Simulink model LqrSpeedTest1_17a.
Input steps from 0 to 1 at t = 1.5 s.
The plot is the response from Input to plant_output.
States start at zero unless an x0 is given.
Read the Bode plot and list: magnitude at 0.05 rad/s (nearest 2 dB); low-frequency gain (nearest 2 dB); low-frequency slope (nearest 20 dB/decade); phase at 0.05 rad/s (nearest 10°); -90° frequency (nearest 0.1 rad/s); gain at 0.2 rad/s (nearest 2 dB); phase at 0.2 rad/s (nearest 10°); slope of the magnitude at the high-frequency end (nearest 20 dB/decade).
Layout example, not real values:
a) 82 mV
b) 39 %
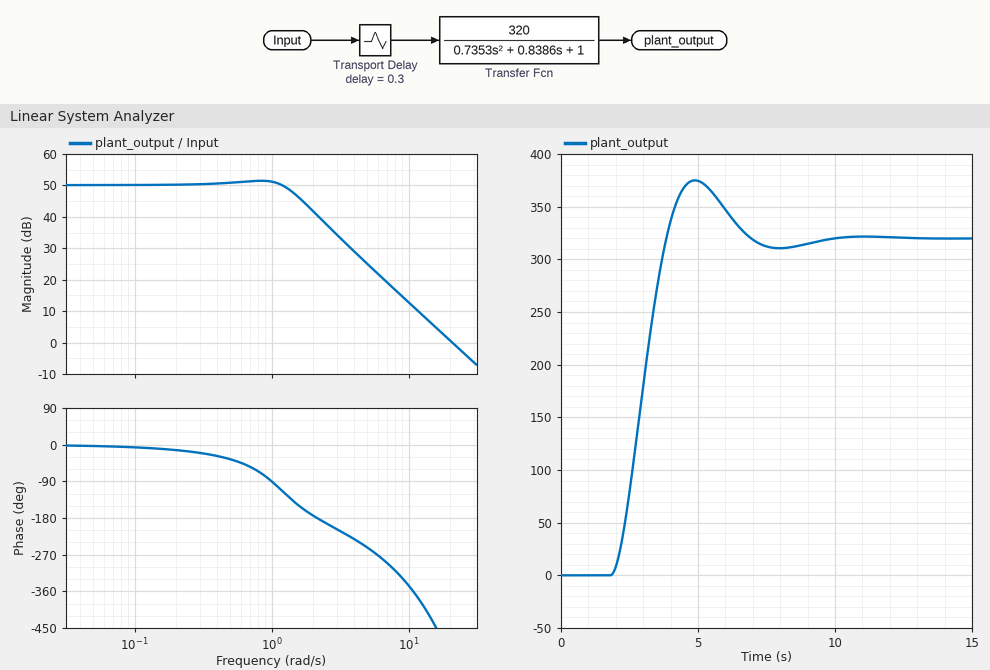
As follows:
a) 50 dB
b) 50 dB
c) 0 dB/decade
d) 0°
e) 1.0 rad/s
f) 50 dB
g) -10°
h) -40 dB/decade
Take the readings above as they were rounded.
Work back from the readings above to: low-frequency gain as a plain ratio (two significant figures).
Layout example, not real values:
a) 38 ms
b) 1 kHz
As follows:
a) 320
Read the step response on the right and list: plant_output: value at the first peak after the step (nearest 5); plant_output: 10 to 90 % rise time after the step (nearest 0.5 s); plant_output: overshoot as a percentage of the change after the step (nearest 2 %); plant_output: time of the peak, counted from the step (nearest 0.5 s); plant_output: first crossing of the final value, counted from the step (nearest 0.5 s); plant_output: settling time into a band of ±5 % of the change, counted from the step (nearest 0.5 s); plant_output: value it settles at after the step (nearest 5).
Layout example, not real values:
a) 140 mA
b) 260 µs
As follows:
a) 375
b) 1.5 s
c) 18 %
d) 3.5 s
e) 2.5 s
f) 5.0 s
g) 320
